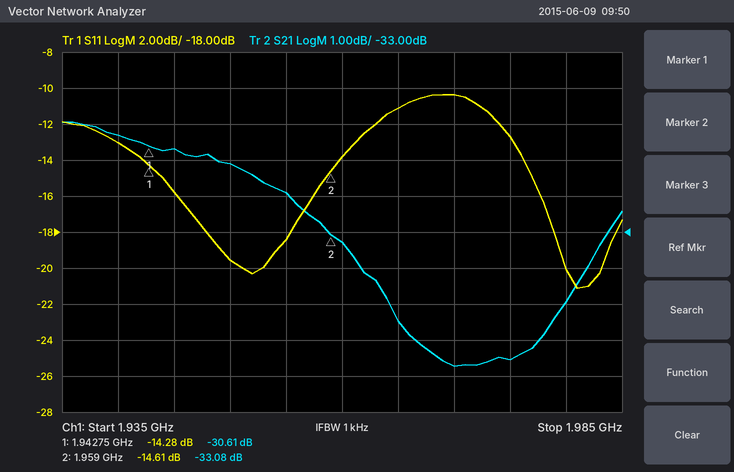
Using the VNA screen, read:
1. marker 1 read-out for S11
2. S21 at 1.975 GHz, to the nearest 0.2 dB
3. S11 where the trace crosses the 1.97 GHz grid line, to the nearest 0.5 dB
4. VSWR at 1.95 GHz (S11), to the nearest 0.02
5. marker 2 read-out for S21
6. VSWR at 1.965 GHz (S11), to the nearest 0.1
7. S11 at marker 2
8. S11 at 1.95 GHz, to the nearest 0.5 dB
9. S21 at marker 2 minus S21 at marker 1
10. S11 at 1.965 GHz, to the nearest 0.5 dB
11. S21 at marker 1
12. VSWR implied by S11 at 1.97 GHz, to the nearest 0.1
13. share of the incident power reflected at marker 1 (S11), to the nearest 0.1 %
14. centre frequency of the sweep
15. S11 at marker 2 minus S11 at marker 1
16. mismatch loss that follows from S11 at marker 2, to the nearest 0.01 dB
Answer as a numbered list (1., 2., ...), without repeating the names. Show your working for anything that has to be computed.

1. -14.28 dB
2. -36.6 dB
3. -10.5 dB
4. |Γ| = 10^(-19.5/20) = 0.1059; VSWR = (1 + 0.1059)/(1 − 0.1059) ≈ 1.24
5. -33.08 dB
6. |Γ| = 10^(-11/20) = 0.2818; VSWR = (1 + 0.2818)/(1 − 0.2818) ≈ 1.8
7. -14.61 dB
8. -19.5 dB
9. -33.08 − (-30.61) = -2.47 dB
10. -11.0 dB
11. -30.61 dB
12. |Γ| = 10^(-10.5/20) = 0.2985; VSWR = (1 + 0.2985)/(1 − 0.2985) ≈ 1.9
13. 10^(-14.28/10) ≈ 3.7 %
14. 1.96 GHz
15. -14.61 − (-14.28) = -0.33 dB
16. −10 log10(1 − 10^(-14.61/10)) ≈ 0.15 dB
